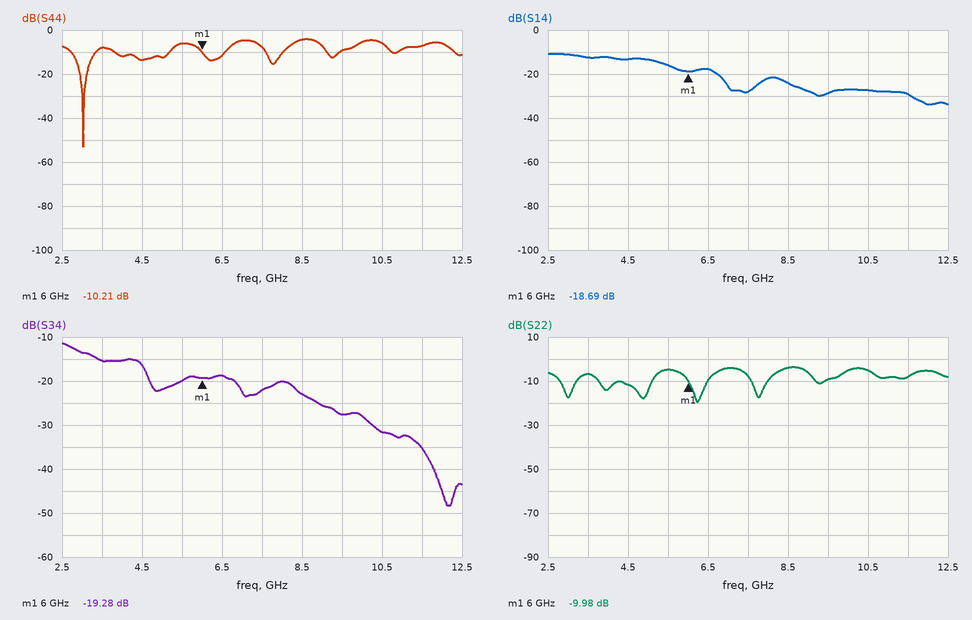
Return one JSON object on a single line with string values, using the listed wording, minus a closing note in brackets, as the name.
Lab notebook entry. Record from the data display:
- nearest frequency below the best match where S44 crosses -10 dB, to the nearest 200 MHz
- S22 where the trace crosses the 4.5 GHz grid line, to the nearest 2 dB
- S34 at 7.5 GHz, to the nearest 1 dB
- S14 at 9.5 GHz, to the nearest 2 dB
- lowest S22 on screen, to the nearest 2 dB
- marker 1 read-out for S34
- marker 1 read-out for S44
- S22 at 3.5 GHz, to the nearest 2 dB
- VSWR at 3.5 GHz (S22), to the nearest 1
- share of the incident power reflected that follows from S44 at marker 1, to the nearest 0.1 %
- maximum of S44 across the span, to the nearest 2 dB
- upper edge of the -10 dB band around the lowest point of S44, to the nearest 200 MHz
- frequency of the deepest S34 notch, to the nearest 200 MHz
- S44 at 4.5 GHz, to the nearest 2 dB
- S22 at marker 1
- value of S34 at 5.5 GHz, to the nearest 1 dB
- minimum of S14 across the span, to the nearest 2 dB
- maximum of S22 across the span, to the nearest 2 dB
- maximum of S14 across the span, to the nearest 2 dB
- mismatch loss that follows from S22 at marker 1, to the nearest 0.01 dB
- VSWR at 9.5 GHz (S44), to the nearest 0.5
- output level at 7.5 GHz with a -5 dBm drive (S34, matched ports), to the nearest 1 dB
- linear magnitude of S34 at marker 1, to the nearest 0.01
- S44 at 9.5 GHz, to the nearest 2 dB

{"nearest frequency below the best match where S44 crosses -10 dB, to the nearest 200 MHz": "2.8 GHz", "S22 where the trace crosses the 4.5 GHz grid line, to the nearest 2 dB": "-12 dB", "S34 at 7.5 GHz, to the nearest 1 dB": "-22 dB", "S14 at 9.5 GHz, to the nearest 2 dB": "-28 dB", "lowest S22 on screen, to the nearest 2 dB": "-20 dB", "marker 1 read-out for S34": "-19.28 dB", "marker 1 read-out for S44": "-10.21 dB", "S22 at 3.5 GHz, to the nearest 2 dB": "-6 dB", "VSWR at 3.5 GHz (S22), to the nearest 1": "3", "share of the incident power reflected that follows from S44 at marker 1, to the nearest 0.1 %": "9.5 %", "maximum of S44 across the span, to the nearest 2 dB": "-4 dB", "upper edge of the -10 dB band around the lowest point of S44, to the nearest 200 MHz": "3.4 GHz", "frequency of the deepest S34 notch, to the nearest 200 MHz": "12.2 GHz", "S44 at 4.5 GHz, to the nearest 2 dB": "-14 dB", "S22 at marker 1": "-9.98 dB", "value of S34 at 5.5 GHz, to the nearest 1 dB": "-20 dB", "minimum of S14 across the span, to the nearest 2 dB": "-34 dB", "maximum of S22 across the span, to the nearest 2 dB": "-4 dB", "maximum of S14 across the span, to the nearest 2 dB": "-10 dB", "mismatch loss that follows from S22 at marker 1, to the nearest 0.01 dB": "0.46 dB", "VSWR at 9.5 GHz (S44), to the nearest 0.5": "2.0", "output level at 7.5 GHz with a -5 dBm drive (S34, matched ports), to the nearest 1 dB": "-27 dBm", "linear magnitude of S34 at marker 1, to the nearest 0.01": "0.11", "S44 at 9.5 GHz, to the nearest 2 dB": "-10 dB"}
